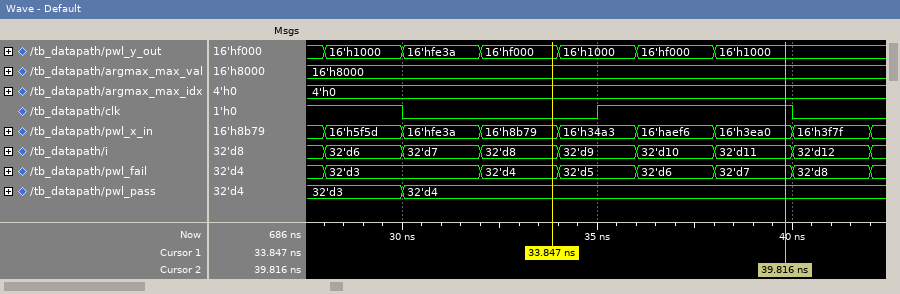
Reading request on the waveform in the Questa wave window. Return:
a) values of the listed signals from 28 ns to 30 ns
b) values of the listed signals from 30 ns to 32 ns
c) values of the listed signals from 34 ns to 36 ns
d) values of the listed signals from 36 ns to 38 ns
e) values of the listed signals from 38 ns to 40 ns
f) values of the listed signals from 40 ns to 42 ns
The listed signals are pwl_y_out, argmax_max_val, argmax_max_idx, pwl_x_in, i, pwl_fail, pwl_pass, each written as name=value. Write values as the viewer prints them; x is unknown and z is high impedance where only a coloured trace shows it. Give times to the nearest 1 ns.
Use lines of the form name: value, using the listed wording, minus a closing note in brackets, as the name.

values of the listed signals from 28 ns to 30 ns: pwl_y_out=16'h1000, argmax_max_val=16'h8000, argmax_max_idx=4'h0, pwl_x_in=16'h5f5d, i=32'd6, pwl_fail=32'd3, pwl_pass=32'd3
values of the listed signals from 30 ns to 32 ns: pwl_y_out=16'hfe3a, argmax_max_val=16'h8000, argmax_max_idx=4'h0, pwl_x_in=16'hfe3a, i=32'd7, pwl_fail=32'd3, pwl_pass=32'd4
values of the listed signals from 34 ns to 36 ns: pwl_y_out=16'h1000, argmax_max_val=16'h8000, argmax_max_idx=4'h0, pwl_x_in=16'h34a3, i=32'd9, pwl_fail=32'd5, pwl_pass=32'd4
values of the listed signals from 36 ns to 38 ns: pwl_y_out=16'hf000, argmax_max_val=16'h8000, argmax_max_idx=4'h0, pwl_x_in=16'haef6, i=32'd10, pwl_fail=32'd6, pwl_pass=32'd4
values of the listed signals from 38 ns to 40 ns: pwl_y_out=16'h1000, argmax_max_val=16'h8000, argmax_max_idx=4'h0, pwl_x_in=16'h3ea0, i=32'd11, pwl_fail=32'd7, pwl_pass=32'd4
values of the listed signals from 40 ns to 42 ns: pwl_y_out=16'h1000, argmax_max_val=16'h8000, argmax_max_idx=4'h0, pwl_x_in=16'h3f7f, i=32'd12, pwl_fail=32'd8, pwl_pass=32'd4
